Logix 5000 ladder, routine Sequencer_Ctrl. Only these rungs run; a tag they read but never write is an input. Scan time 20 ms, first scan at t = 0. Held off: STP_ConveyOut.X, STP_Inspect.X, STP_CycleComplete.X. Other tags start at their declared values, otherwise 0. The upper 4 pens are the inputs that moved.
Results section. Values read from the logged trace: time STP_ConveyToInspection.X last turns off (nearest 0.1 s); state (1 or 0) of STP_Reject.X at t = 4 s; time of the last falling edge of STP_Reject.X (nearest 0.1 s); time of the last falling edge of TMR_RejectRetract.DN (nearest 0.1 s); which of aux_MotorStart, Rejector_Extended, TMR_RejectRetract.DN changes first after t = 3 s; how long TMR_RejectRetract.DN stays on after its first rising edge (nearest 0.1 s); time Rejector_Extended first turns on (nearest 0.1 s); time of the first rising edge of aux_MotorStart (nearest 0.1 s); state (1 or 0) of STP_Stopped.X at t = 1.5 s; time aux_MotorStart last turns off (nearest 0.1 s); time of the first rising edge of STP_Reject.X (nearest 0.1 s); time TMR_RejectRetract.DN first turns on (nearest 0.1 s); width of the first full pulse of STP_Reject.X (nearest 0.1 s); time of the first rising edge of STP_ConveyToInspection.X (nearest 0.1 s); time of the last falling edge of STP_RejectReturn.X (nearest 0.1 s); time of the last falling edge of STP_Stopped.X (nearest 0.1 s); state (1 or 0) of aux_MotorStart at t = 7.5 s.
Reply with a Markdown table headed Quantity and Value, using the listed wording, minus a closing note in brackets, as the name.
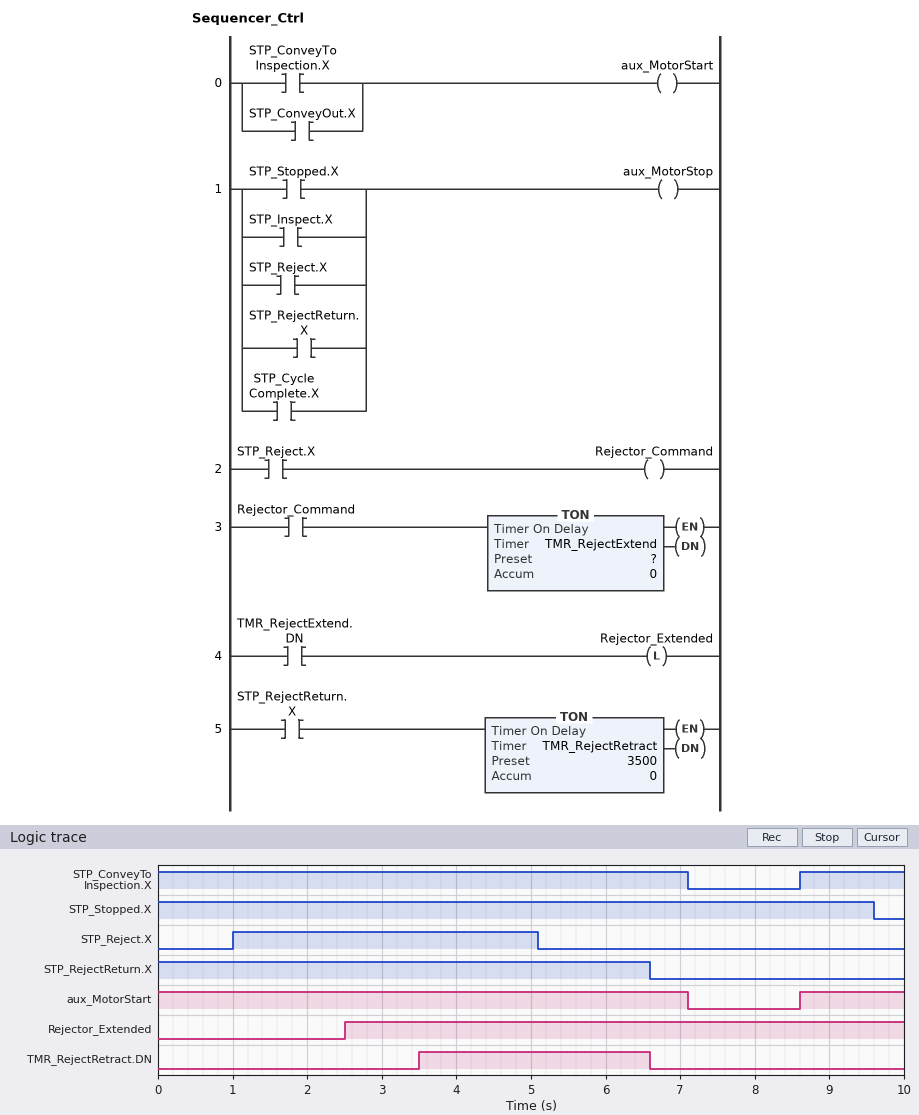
| Quantity | Value |
|---|---|
| time STP_ConveyToInspection.X last turns off | 7.1 s |
| state (1 or 0) of STP_Reject.X at t = 4 s | 1 |
| time of the last falling edge of STP_Reject.X | 5.1 s |
| time of the last falling edge of TMR_RejectRetract.DN | 6.6 s |
| which of aux_MotorStart, Rejector_Extended, TMR_RejectRetract.DN changes first after t = 3 s | TMR_RejectRetract.DN |
| how long TMR_RejectRetract.DN stays on after its first rising edge | 3.1 s |
| time Rejector_Extended first turns on | 2.5 s |
| time of the first rising edge of aux_MotorStart | 8.6 s |
| state (1 or 0) of STP_Stopped.X at t = 1.5 s | 1 |
| time aux_MotorStart last turns off | 7.1 s |
| time of the first rising edge of STP_Reject.X | 1.0 s |
| time TMR_RejectRetract.DN first turns on | 3.5 s |
| width of the first full pulse of STP_Reject.X | 4.1 s |
| time of the first rising edge of STP_ConveyToInspection.X | 8.6 s |
| time of the last falling edge of STP_RejectReturn.X | 6.6 s |
| time of the last falling edge of STP_Stopped.X | 9.6 s |
| state (1 or 0) of aux_MotorStart at t = 7.5 s | 0 |
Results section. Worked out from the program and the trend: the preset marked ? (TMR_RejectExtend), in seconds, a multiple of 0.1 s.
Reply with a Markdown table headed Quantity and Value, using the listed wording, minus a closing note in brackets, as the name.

| Quantity | Value |
|---|---|
| the preset marked ? (TMR_RejectExtend), in seconds, a multiple of 0.1 s | 1.5 s |
